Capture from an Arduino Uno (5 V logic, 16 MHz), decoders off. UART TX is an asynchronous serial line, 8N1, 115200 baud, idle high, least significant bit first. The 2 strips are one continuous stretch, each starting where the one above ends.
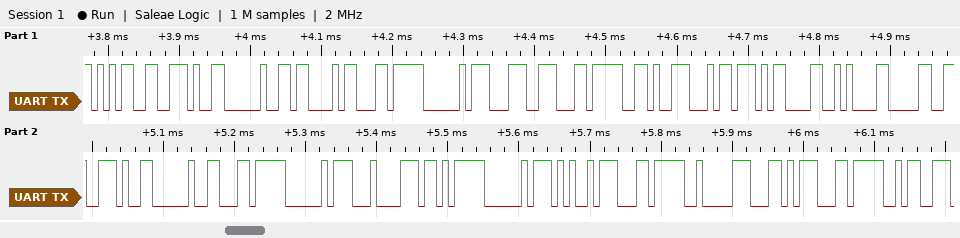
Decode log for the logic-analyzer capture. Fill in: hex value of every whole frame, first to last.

35 2E 20 43 EC A0 9C EC 96 B4 0D 0A 30 2E 20 EC A0 84 EB A0 A5 EC 82 AC EC 9A
